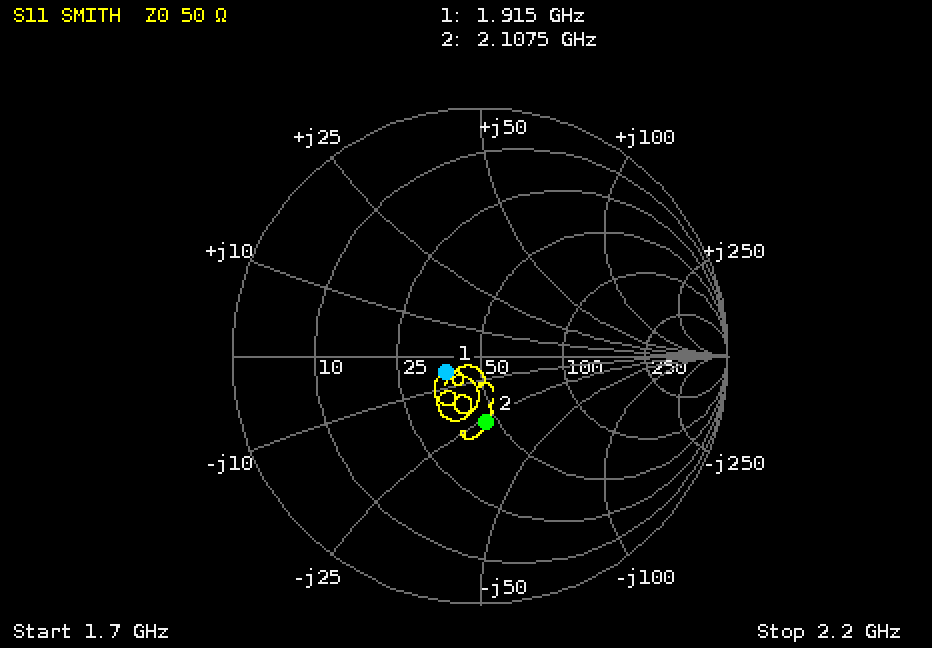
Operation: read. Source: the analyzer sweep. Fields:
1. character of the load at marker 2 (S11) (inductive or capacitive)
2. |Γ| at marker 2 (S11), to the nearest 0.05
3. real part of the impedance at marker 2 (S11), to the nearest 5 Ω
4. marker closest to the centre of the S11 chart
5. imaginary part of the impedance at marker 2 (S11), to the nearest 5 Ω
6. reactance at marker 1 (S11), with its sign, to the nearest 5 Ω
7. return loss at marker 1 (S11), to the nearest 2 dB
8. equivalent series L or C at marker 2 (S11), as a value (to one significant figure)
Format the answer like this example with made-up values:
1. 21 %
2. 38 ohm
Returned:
1. capacitive
2. 0.25
3. 45 Ω
4. marker 1
5. -25 Ω
6. -5 Ω
7. 16 dB
8. 3 pF
